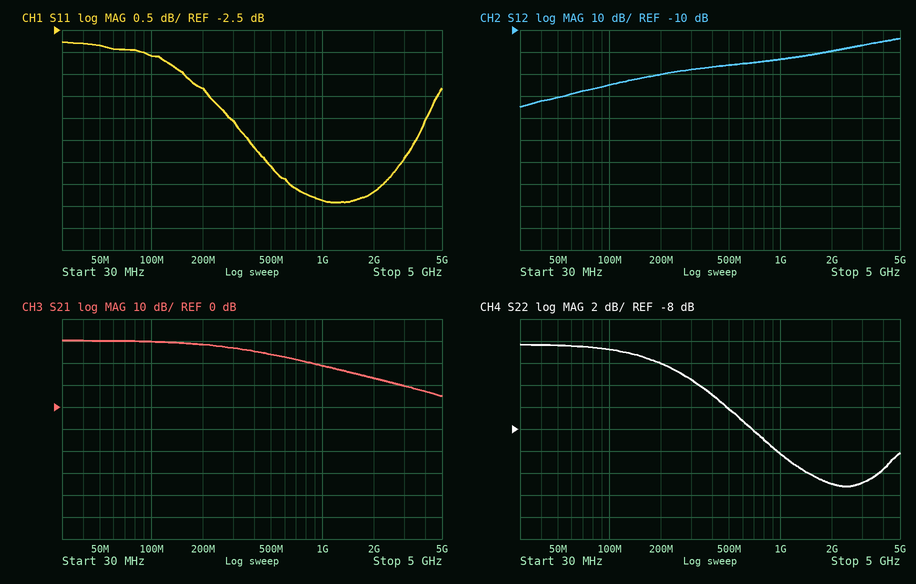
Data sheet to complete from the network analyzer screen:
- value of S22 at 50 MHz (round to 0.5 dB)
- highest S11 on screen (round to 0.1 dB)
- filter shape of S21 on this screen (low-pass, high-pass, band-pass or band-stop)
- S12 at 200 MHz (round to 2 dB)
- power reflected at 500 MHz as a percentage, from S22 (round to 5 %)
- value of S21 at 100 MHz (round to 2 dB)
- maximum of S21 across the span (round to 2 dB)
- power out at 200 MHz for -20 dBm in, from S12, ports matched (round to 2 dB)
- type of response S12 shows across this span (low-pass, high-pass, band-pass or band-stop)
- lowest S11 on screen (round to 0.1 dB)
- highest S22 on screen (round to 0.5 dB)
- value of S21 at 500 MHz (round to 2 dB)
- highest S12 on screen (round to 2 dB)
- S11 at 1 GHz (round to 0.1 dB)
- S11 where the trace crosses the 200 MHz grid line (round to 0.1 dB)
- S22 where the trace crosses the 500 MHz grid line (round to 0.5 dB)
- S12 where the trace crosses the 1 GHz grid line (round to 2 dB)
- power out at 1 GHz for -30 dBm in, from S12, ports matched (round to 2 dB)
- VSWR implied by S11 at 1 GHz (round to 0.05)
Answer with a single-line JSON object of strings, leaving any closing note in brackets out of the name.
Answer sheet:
{"value of S22 at 50 MHz": "-0.5 dB", "highest S11 on screen": "-2.8 dB", "filter shape of S21 on this screen": "low-pass", "S12 at 200 MHz": "-30 dB", "power reflected at 500 MHz as a percentage, from S22": "25 %", "value of S21 at 100 MHz": "30 dB", "maximum of S21 across the span": "30 dB", "power out at 200 MHz for -20 dBm in, from S12, ports matched": "-50 dBm", "type of response S12 shows across this span": "high-pass", "lowest S11 on screen": "-6.4 dB", "highest S22 on screen": "-0.5 dB", "value of S21 at 500 MHz": "24 dB", "highest S12 on screen": "-14 dB", "S11 at 1 GHz": "-6.4 dB", "S11 where the trace crosses the 200 MHz grid line": "-3.8 dB", "S22 where the trace crosses the 500 MHz grid line": "-6.0 dB", "S12 where the trace crosses the 1 GHz grid line": "-24 dB", "power out at 1 GHz for -30 dBm in, from S12, ports matched": "-54 dBm", "VSWR implied by S11 at 1 GHz": "2.85"}
